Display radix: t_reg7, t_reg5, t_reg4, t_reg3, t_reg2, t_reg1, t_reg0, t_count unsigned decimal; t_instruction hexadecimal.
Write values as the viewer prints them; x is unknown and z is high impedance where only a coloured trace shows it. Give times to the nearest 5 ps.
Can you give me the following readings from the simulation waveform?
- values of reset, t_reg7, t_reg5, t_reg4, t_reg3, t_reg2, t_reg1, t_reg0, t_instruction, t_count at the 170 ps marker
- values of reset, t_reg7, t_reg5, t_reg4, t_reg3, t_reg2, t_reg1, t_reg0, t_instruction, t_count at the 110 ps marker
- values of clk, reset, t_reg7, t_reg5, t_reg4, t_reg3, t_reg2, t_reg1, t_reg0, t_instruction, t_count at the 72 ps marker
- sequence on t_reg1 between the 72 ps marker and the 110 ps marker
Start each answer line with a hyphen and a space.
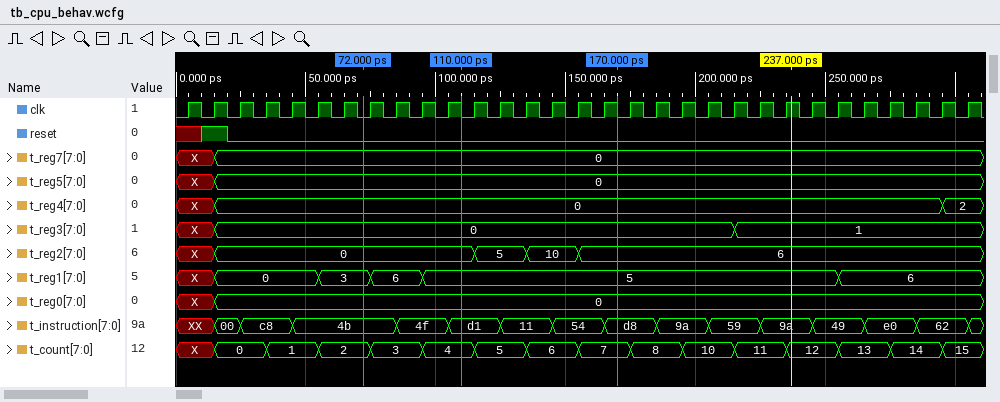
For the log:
- reset=0, t_reg7=0, t_reg5=0, t_reg4=0, t_reg3=0, t_reg2=6, t_reg1=5, t_reg0=0, t_instruction=d8, t_count=7
- reset=0, t_reg7=0, t_reg5=0, t_reg4=0, t_reg3=0, t_reg2=0, t_reg1=5, t_reg0=0, t_instruction=d1, t_count=4
- clk=0, reset=0, t_reg7=0, t_reg5=0, t_reg4=0, t_reg3=0, t_reg2=0, t_reg1=3, t_reg0=0, t_instruction=4b, t_count=2
- 3, 6, 5
